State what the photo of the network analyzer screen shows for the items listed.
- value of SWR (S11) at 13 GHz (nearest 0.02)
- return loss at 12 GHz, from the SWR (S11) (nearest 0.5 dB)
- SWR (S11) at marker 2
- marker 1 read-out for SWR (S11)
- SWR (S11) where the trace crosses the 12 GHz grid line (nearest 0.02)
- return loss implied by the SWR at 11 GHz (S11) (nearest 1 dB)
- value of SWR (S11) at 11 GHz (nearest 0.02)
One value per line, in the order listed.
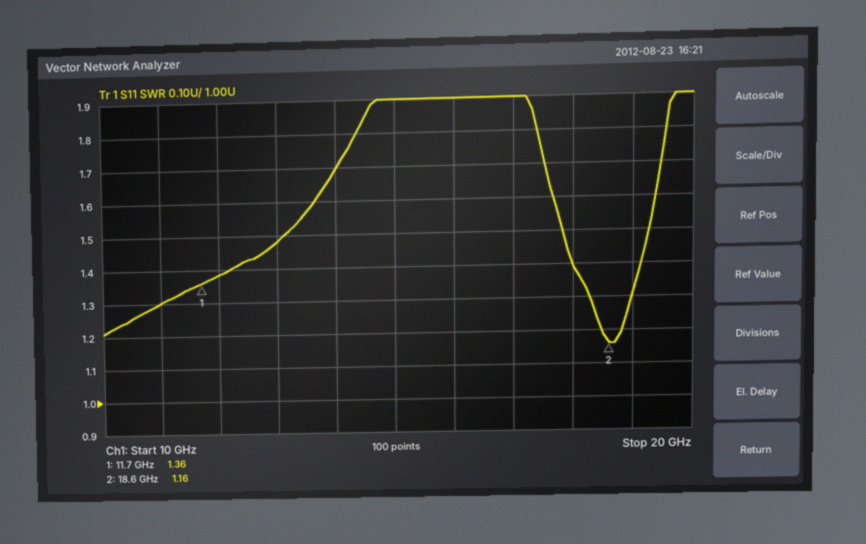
1.48
16.0 dB
1.16
1.36
1.38
18 dB
1.30
